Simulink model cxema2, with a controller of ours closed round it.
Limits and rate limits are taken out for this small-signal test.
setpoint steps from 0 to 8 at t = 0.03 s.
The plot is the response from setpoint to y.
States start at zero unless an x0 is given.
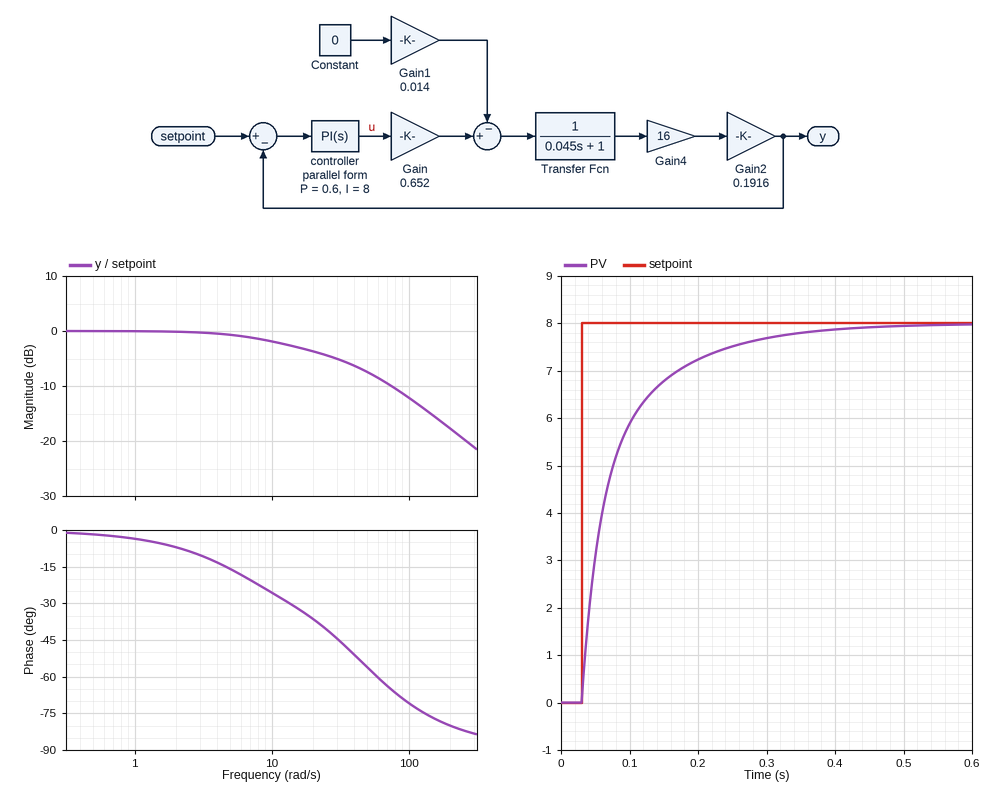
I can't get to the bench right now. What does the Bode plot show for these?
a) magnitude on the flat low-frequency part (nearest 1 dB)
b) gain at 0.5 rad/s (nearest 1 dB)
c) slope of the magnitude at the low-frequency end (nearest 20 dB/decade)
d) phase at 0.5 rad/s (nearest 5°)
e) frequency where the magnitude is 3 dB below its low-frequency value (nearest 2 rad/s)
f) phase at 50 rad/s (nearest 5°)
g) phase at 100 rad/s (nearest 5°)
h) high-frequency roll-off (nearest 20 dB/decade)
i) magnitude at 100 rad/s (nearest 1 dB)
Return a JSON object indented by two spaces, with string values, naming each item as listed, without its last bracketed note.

{
  "magnitude on the flat low-frequency part": "0 dB",
  "gain at 0.5 rad/s": "0 dB",
  "slope of the magnitude at the low-frequency end": "0 dB/decade",
  "phase at 0.5 rad/s": "0°",
  "frequency where the magnitude is 3 dB below its low-frequency value": "16 rad/s",
  "phase at 50 rad/s": "-55°",
  "phase at 100 rad/s": "-70°",
  "high-frequency roll-off": "-20 dB/decade",
  "magnitude at 100 rad/s": "-12 dB"
}
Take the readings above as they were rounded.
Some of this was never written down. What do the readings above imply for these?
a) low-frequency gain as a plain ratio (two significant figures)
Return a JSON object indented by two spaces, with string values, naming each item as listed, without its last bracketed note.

{
  "low-frequency gain as a plain ratio": "1.0"
}
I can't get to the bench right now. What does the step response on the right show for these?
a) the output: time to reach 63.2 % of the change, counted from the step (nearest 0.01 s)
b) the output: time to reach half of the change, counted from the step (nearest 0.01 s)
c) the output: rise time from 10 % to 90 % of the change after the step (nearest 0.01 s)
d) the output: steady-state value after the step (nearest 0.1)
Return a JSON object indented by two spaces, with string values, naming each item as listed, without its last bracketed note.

{
  "the output: time to reach 63.2 % of the change, counted from the step": "0.05 s",
  "the output: time to reach half of the change, counted from the step": "0.03 s",
  "the output: rise time from 10 % to 90 % of the change after the step": "0.16 s",
  "the output: steady-state value after the step": "8.0"
}
